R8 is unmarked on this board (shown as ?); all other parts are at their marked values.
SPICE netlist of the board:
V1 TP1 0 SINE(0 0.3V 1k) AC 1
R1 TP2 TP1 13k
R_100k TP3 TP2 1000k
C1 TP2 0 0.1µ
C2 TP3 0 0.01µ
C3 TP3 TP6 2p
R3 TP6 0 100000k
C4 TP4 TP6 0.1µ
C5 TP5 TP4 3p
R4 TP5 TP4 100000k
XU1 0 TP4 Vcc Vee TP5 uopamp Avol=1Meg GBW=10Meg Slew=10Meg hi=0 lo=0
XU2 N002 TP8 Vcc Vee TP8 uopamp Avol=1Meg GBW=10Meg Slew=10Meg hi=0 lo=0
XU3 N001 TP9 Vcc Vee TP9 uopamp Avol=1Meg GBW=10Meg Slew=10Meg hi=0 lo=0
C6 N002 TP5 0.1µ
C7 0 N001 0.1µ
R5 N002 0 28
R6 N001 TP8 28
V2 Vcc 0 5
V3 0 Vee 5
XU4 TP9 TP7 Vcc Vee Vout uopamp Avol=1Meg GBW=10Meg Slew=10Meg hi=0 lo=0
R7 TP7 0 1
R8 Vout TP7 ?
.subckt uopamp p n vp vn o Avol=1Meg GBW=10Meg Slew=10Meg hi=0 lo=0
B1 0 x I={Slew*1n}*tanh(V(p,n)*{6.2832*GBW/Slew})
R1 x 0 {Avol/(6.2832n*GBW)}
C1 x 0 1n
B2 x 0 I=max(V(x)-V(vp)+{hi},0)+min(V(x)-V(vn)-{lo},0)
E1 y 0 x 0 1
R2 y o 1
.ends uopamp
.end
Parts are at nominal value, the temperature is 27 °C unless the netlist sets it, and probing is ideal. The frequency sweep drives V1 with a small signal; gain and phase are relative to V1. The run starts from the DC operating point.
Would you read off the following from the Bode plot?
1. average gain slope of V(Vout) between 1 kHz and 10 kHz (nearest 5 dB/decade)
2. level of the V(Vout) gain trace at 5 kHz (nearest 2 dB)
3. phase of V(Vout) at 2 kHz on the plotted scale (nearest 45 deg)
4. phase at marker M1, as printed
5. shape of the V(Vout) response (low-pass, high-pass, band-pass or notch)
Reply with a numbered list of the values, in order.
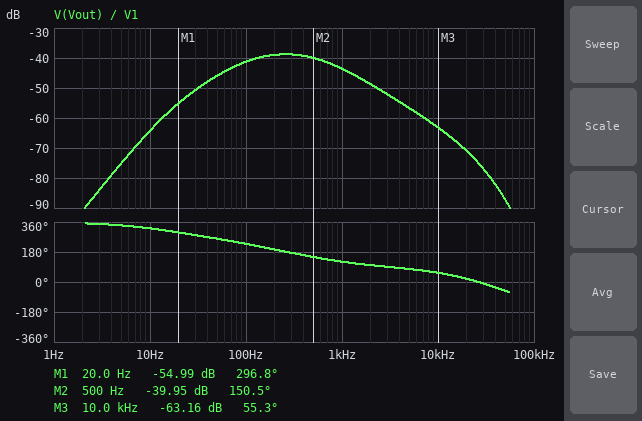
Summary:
1. -20 dB/decade
2. -56 dB
3. 90 deg
4. 296.8 deg
5. band-pass
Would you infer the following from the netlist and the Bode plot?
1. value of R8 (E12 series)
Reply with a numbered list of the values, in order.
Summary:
1. 330 Ω
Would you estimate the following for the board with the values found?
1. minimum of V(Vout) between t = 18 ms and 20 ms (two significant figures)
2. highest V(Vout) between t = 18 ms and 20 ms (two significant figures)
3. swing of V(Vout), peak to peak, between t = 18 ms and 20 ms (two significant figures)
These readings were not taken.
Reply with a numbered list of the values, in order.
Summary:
1. -2.0 mV
2. 2.0 mV
3. 4.0 mV
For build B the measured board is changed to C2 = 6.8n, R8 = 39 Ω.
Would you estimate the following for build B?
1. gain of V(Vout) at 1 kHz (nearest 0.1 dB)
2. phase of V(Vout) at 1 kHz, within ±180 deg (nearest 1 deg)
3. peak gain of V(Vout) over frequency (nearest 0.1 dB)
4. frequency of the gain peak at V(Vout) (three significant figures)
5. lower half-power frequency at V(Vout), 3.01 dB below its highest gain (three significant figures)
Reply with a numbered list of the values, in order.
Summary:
1. -58.6 dB
2. 124 deg
3. -53.8 dB
4. 260 Hz
5. 92.5 Hz
